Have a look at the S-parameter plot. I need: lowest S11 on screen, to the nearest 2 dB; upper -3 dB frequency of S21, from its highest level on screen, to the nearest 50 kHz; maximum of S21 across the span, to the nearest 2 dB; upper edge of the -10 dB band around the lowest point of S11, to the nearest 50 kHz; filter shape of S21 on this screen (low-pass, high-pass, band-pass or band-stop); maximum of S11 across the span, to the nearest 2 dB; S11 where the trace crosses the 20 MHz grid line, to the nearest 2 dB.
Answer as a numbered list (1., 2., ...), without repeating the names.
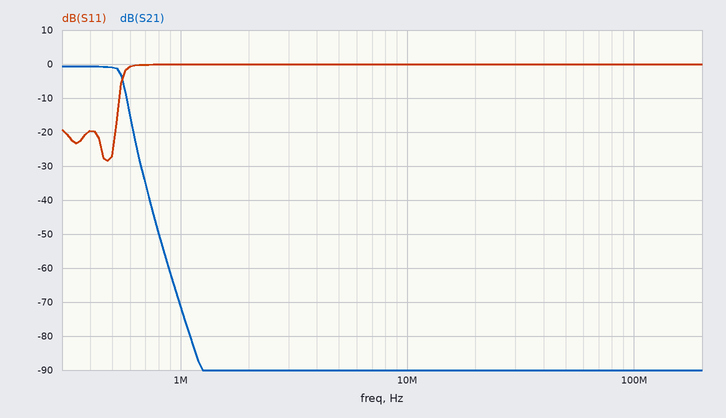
1. -28 dB
2. 550 kHz
3. 0 dB
4. 550 kHz
5. low-pass
6. 0 dB
7. 0 dB
